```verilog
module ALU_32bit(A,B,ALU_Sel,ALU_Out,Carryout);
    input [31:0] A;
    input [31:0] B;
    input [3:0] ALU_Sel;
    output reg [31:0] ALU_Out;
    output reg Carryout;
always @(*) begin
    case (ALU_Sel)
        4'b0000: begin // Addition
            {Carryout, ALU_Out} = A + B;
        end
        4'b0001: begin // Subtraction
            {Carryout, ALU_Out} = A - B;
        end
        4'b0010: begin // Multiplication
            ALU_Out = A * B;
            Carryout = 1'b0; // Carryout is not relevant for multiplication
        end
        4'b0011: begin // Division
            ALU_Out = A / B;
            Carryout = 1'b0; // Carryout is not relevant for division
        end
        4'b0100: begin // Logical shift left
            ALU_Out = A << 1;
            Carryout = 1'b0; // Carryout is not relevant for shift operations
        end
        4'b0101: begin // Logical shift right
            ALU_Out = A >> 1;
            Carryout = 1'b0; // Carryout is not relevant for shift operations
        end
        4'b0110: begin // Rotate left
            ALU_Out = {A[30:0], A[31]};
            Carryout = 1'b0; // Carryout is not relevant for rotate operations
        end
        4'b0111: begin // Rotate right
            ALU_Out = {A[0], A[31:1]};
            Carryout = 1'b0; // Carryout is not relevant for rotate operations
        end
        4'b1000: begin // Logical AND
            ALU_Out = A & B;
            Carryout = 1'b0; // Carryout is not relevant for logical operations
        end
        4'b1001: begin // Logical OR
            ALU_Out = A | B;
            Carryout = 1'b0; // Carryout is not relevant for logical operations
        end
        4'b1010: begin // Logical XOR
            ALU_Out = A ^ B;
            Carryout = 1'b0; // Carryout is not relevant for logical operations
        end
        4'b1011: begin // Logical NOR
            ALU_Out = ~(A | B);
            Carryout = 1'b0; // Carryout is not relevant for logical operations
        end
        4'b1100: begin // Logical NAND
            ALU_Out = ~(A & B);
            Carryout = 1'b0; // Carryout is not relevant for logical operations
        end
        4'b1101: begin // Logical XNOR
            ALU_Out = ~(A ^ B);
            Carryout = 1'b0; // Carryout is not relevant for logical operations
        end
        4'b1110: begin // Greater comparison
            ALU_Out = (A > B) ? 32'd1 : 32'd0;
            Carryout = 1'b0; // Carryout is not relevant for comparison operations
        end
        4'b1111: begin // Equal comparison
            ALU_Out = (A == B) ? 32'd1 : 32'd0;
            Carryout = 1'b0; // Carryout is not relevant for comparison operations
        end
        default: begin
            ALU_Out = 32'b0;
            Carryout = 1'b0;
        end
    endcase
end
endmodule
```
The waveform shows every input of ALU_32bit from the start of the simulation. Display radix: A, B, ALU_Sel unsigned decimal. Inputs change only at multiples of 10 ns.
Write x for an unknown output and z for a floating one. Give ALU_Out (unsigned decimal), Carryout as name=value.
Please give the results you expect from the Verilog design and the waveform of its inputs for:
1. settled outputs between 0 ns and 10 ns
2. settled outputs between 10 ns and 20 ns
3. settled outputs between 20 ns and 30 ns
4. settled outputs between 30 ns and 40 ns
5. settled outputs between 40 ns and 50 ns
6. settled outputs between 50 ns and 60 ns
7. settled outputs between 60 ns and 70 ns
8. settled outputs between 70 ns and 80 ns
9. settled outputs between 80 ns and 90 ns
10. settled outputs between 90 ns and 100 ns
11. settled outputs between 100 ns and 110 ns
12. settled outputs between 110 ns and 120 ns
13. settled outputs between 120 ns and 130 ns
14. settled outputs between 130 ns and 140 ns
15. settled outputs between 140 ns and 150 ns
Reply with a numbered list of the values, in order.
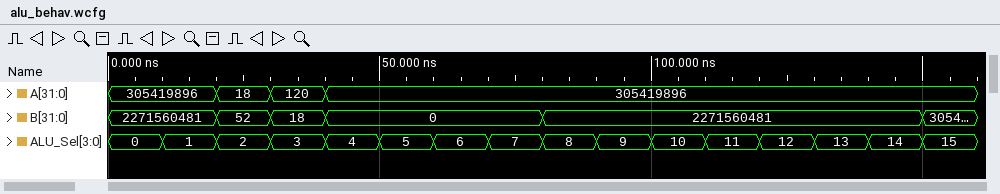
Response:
1. ALU_Out=2576980377, Carryout=0
2. ALU_Out=2328826711, Carryout=1
3. ALU_Out=936, Carryout=0
4. ALU_Out=6, Carryout=0
5. ALU_Out=610839792, Carryout=0
6. ALU_Out=152709948, Carryout=0
7. ALU_Out=610839792, Carryout=0
8. ALU_Out=152709948, Carryout=0
9. ALU_Out=35930656, Carryout=0
10. ALU_Out=2541049721, Carryout=0
11. ALU_Out=2505119065, Carryout=0
12. ALU_Out=1753917574, Carryout=0
13. ALU_Out=4259036639, Carryout=0
14. ALU_Out=1789848230, Carryout=0
15. ALU_Out=0, Carryout=0
